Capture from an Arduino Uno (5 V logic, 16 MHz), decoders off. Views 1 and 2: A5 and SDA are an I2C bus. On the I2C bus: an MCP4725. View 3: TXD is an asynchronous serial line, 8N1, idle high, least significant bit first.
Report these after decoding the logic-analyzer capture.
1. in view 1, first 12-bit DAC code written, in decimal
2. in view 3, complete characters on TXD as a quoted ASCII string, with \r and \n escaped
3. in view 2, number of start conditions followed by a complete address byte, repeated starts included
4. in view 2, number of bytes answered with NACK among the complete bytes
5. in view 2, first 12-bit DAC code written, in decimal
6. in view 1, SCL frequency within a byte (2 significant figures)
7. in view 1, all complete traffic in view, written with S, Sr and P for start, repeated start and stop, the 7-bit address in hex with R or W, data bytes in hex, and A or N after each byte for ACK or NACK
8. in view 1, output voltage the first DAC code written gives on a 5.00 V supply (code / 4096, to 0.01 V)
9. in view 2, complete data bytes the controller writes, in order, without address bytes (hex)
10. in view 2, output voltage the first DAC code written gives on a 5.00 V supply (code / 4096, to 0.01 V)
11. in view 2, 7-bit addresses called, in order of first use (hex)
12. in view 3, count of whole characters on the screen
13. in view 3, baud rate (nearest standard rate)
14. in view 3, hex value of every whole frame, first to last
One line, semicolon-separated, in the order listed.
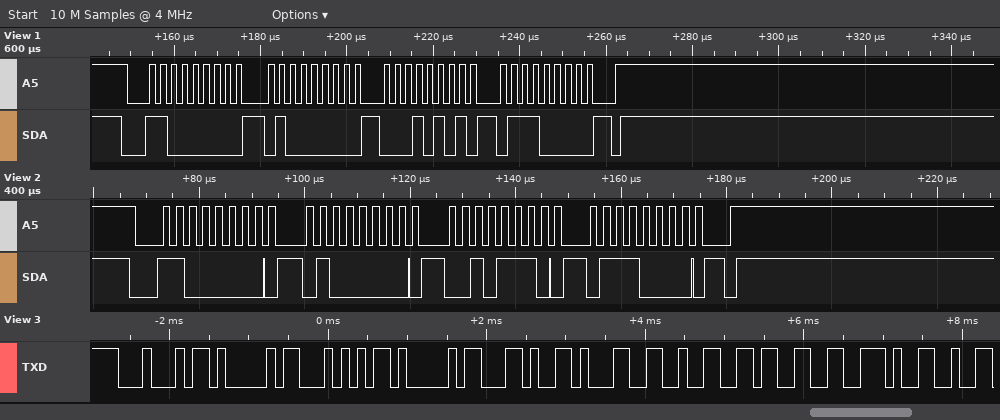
343; "DATA,123."; 1; 0; 743; 400 kHz; S 60W A 40 A 15 A 70 A P; 0.42 V; 40 2E 70; 0.91 V; 0x60; 9; 9600 baud; 44 41 54 41 2C 31 32 33 2E
